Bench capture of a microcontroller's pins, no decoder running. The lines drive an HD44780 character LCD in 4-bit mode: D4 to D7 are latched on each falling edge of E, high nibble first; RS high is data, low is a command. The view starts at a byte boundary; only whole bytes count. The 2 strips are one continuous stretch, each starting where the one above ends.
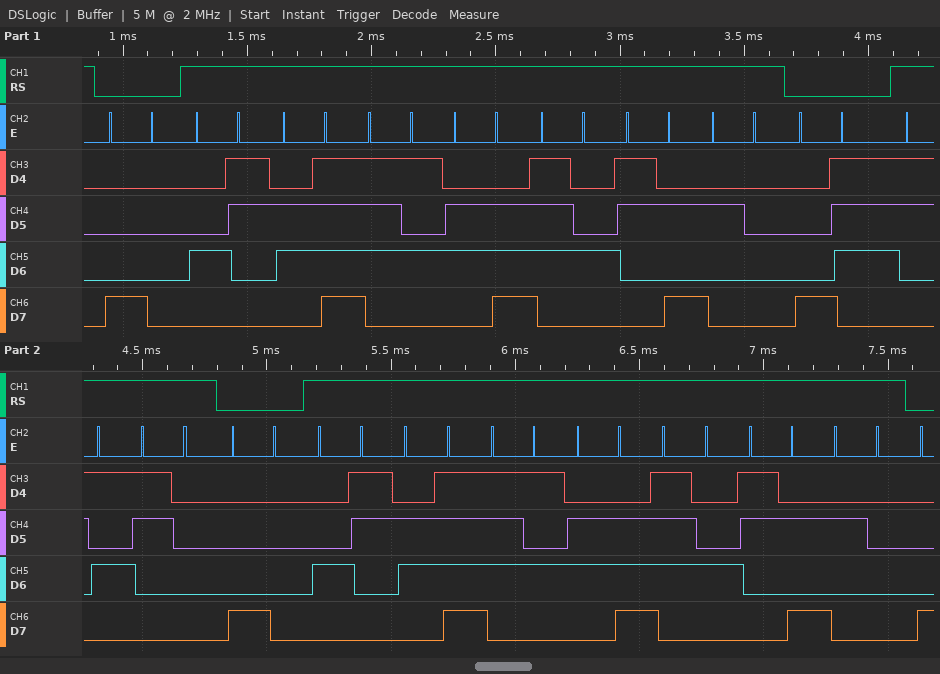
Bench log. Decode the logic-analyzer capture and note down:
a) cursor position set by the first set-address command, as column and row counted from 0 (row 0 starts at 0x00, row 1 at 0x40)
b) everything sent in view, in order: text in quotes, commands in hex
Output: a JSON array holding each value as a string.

["column 0, row 0", "0x80 \"Count: \" 0x87 \"50\" 0x80 \"Count: \""]
